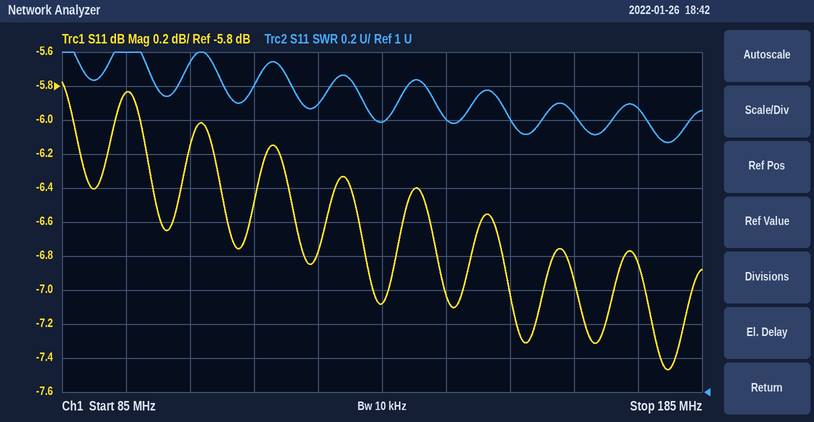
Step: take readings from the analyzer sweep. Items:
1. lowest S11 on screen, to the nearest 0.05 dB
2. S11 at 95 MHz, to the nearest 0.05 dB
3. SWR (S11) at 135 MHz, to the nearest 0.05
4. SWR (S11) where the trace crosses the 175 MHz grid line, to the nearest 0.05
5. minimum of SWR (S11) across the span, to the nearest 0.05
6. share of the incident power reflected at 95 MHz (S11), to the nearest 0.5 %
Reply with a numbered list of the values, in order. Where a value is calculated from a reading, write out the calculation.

1. -7.45 dB
2. -5.85 dB
3. 2.60
4. 2.65
5. 2.45
6. 10^(-5.85/10) ≈ 26.0 %
